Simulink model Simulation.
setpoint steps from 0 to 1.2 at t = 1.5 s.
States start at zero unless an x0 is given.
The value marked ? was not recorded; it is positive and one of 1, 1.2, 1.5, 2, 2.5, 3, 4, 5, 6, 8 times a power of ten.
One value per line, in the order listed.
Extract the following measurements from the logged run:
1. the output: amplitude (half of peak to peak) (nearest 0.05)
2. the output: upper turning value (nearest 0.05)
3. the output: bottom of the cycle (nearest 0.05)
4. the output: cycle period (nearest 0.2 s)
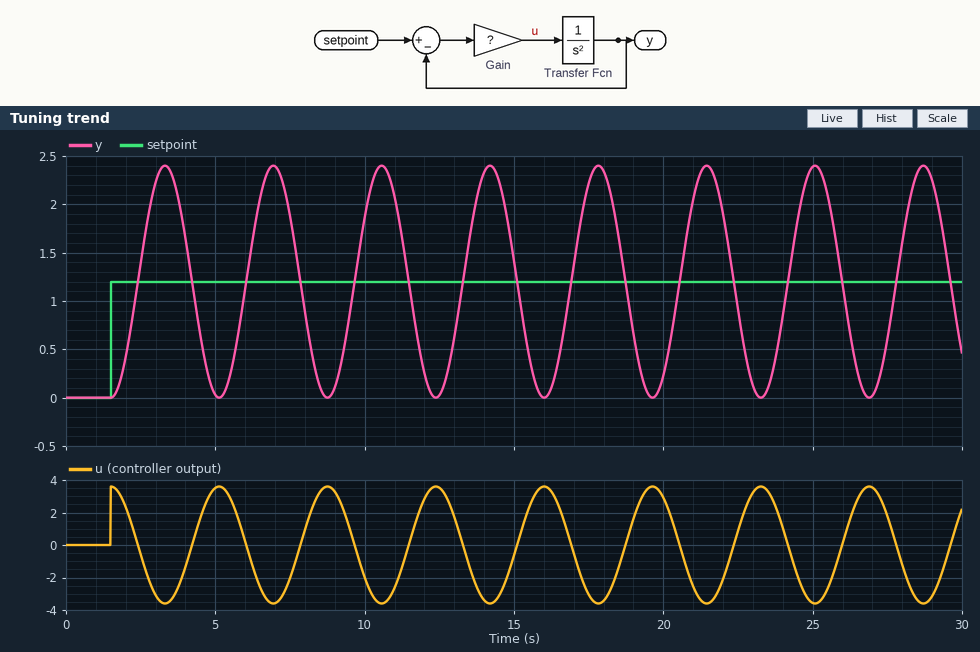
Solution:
1.20
2.40
0.00
3.6 s
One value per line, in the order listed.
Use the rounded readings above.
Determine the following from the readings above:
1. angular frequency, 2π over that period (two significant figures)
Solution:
1.7 rad/s
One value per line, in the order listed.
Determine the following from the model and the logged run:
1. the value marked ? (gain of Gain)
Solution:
3
